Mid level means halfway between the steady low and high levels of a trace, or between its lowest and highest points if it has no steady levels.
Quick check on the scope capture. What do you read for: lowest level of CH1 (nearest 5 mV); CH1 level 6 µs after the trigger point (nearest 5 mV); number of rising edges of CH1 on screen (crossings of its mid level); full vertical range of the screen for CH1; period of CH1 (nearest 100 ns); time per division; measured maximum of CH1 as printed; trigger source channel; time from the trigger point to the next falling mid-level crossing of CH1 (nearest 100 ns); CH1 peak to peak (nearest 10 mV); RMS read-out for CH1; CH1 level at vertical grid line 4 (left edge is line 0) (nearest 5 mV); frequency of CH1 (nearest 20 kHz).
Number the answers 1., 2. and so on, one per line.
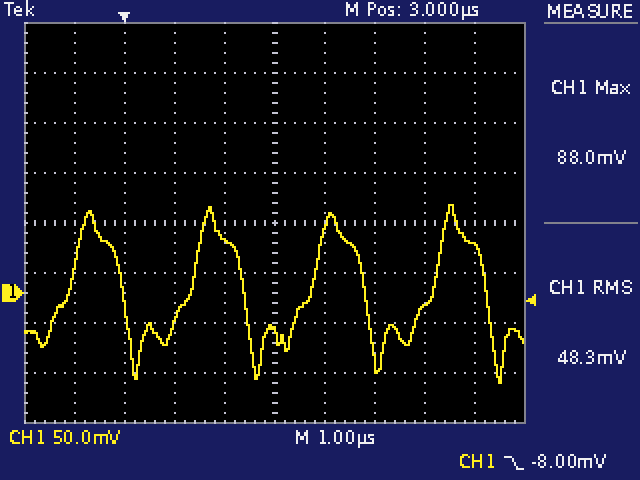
1. -90 mV
2. -15 mV
3. 4
4. 400 mV
5. 2.4 µs
6. 1 µs
7. 88.0 mV
8. CH1
9. 2.4 µs
10. 180 mV
11. 48.3 mV
12. 55 mV
13. 420 kHz
